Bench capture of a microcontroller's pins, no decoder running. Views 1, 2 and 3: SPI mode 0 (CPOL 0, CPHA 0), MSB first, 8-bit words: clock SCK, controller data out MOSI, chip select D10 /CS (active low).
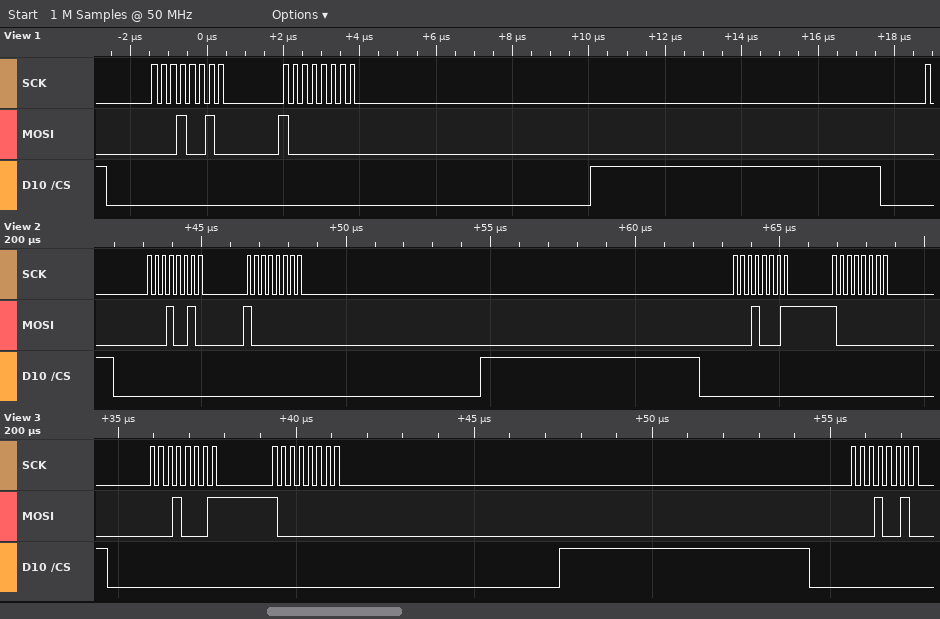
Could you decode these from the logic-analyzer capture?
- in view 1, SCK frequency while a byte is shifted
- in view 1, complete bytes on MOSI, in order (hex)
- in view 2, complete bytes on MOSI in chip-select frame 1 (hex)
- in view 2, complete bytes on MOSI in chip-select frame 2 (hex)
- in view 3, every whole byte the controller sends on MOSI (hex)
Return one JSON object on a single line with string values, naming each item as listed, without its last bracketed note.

{"in view 1, SCK frequency while a byte is shifted": "4 MHz", "in view 1, complete bytes on MOSI, in order": "12 80", "in view 2, complete bytes on MOSI in chip-select frame 1": "0x12 0x80", "in view 2, complete bytes on MOSI in chip-select frame 2": "0x11 0x80", "in view 3, every whole byte the controller sends on MOSI": "11 80 12"}
